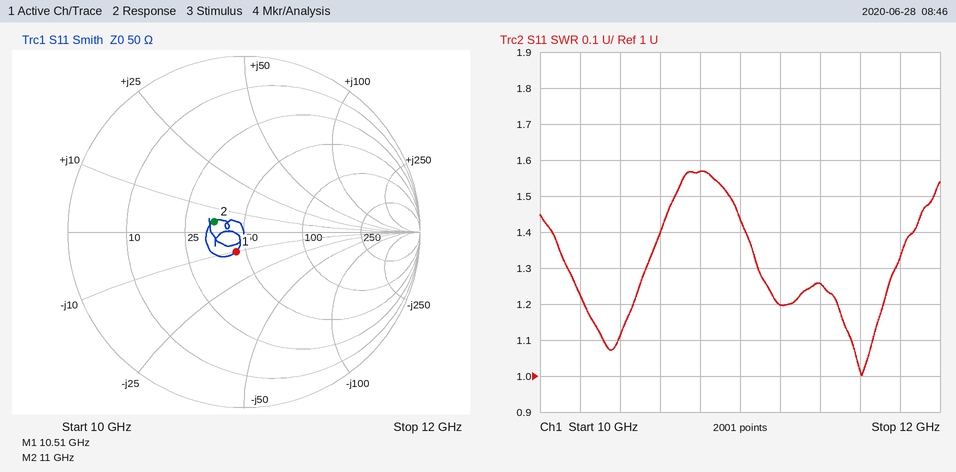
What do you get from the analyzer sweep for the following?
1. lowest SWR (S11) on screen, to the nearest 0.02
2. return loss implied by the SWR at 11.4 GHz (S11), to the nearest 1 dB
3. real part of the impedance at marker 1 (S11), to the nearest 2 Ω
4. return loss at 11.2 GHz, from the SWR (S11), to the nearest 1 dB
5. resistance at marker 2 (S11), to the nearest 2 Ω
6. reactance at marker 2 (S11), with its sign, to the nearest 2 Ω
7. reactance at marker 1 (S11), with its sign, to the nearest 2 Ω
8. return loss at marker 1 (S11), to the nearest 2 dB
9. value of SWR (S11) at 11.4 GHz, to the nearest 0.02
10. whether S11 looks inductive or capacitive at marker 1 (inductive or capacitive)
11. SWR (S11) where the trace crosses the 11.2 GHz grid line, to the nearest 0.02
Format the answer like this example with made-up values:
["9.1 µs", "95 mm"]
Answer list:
["1.00", "19 dB", "44 Ω", "21 dB", "36 Ω", "+4 Ω", "-10 Ω", "18 dB", "1.26", "capacitive", "1.20"]
